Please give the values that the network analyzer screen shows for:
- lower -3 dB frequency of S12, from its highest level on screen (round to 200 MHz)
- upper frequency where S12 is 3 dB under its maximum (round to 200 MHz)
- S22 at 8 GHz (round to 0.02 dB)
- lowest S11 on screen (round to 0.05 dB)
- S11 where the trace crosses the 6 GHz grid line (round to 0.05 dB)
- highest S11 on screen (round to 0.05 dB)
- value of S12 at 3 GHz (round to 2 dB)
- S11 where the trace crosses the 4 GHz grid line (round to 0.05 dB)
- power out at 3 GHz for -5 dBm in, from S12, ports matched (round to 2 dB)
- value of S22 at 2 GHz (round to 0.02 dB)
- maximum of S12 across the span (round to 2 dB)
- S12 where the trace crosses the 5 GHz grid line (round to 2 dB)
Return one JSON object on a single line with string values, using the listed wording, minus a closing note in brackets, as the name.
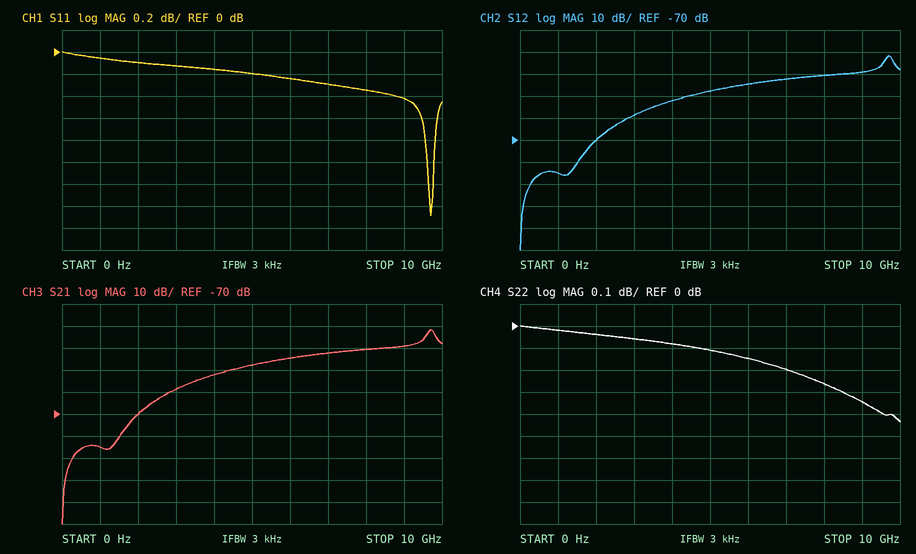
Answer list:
{"lower -3 dB frequency of S12, from its highest level on screen": "9.6 GHz", "upper frequency where S12 is 3 dB under its maximum": "9.8 GHz", "S22 at 8 GHz": "-0.26 dB", "lowest S11 on screen": "-1.50 dB", "S11 where the trace crosses the 6 GHz grid line": "-0.25 dB", "highest S11 on screen": "0.00 dB", "value of S12 at 3 GHz": "-58 dB", "S11 where the trace crosses the 4 GHz grid line": "-0.15 dB", "power out at 3 GHz for -5 dBm in, from S12, ports matched": "-64 dBm", "value of S22 at 2 GHz": "-0.04 dB", "maximum of S12 across the span": "-32 dB", "S12 where the trace crosses the 5 GHz grid line": "-48 dB"}
